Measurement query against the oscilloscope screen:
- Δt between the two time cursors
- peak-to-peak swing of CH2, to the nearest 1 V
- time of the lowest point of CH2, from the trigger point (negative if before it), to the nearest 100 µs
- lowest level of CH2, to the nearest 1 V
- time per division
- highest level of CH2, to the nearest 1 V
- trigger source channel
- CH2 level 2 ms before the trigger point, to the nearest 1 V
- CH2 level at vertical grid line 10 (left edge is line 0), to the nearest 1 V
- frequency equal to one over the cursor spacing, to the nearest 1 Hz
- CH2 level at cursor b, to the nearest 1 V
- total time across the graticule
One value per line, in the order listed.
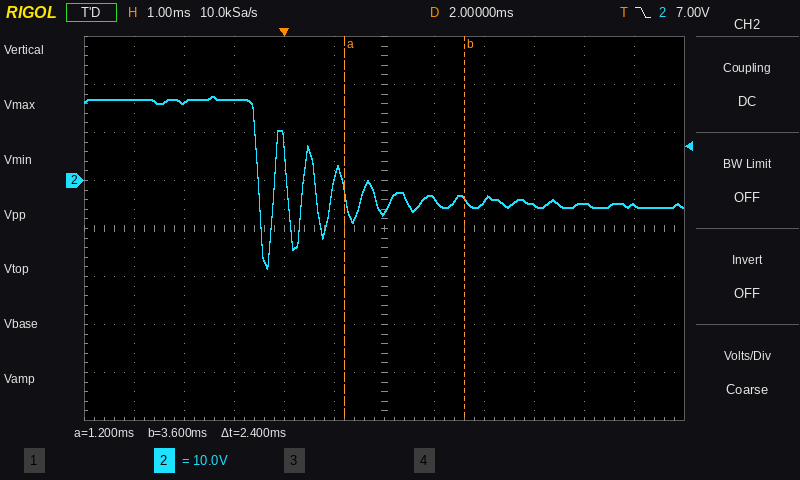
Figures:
2.4 ms
36 V
-300 µs
-18 V
1 ms
18 V
CH2
16 V
-5 V
417 Hz
-4 V
12 ms
